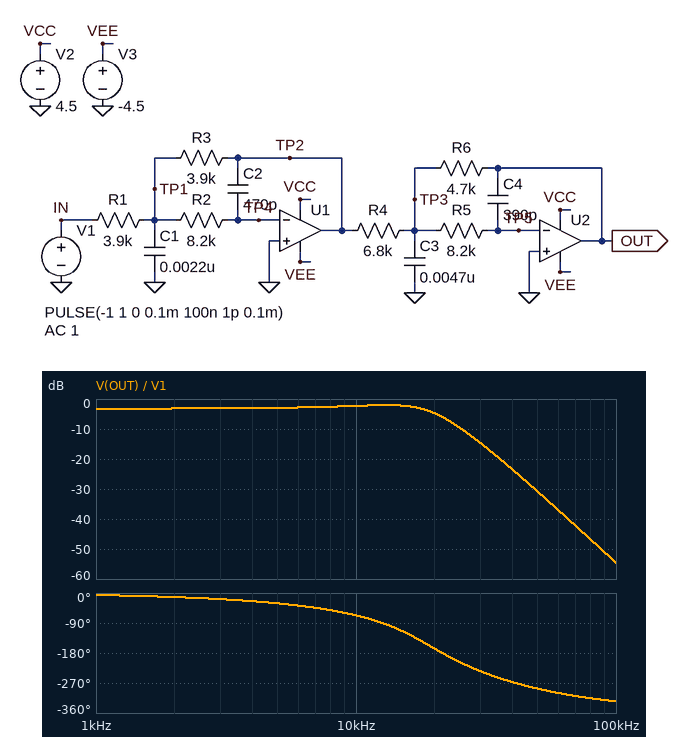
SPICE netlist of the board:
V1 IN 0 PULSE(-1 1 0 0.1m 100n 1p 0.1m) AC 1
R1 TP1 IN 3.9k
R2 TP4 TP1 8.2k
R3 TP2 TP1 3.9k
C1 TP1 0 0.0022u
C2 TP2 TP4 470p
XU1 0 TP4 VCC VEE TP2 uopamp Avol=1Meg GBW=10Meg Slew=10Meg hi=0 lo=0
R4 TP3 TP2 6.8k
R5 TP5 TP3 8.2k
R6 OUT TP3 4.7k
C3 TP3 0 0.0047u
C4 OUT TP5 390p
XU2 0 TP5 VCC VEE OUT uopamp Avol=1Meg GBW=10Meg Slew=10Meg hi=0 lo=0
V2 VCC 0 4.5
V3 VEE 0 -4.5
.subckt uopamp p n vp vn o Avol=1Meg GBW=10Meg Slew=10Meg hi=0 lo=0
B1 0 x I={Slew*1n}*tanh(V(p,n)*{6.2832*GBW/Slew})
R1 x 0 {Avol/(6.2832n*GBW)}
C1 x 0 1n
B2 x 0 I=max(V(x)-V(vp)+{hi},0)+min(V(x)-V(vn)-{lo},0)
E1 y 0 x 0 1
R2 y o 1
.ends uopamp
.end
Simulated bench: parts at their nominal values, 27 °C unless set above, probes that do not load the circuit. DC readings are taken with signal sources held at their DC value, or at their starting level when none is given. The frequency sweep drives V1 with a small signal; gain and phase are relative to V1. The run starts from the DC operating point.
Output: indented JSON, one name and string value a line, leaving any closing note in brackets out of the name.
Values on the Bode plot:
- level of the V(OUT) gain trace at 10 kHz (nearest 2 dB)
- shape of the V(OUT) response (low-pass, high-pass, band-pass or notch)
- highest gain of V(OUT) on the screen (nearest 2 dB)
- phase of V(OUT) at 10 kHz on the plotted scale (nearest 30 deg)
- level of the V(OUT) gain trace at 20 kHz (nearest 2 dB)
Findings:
{
  "level of the V(OUT) gain trace at 10 kHz": "-2 dB",
  "shape of the V(OUT) response": "low-pass",
  "highest gain of V(OUT) on the screen": "-2 dB",
  "phase of V(OUT) at 10 kHz on the plotted scale": "-60 deg",
  "level of the V(OUT) gain trace at 20 kHz": "-4 dB"
}
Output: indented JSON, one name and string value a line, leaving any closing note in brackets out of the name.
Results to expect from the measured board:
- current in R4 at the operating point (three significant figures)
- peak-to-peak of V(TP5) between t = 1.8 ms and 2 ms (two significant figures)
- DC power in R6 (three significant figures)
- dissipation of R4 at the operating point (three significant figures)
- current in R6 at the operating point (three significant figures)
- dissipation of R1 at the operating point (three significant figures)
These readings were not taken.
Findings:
{
  "current in R4 at the operating point": "147 µA",
  "peak-to-peak of V(TP5) between t = 1.8 ms and 2 ms": "1.5 mV",
  "DC power in R6": "102 µW",
  "dissipation of R4 at the operating point": "147 µW",
  "current in R6 at the operating point": "147 µA",
  "dissipation of R1 at the operating point": "256 µW"
}
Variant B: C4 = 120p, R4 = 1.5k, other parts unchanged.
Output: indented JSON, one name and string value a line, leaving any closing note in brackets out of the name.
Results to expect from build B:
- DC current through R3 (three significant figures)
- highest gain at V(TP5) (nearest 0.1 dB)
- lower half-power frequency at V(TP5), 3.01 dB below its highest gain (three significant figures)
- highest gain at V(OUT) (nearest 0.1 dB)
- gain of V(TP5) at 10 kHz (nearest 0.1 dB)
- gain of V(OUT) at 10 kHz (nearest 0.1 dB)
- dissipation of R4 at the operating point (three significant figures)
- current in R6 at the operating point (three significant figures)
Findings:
{
  "DC current through R3": "256 µA",
  "highest gain at V(TP5)": "-44.4 dB",
  "lower half-power frequency at V(TP5), 3.01 dB below its highest gain": "14.1 kHz",
  "highest gain at V(OUT)": "9.9 dB",
  "gain of V(TP5) at 10 kHz": "-50.2 dB",
  "gain of V(OUT) at 10 kHz": "9.8 dB",
  "dissipation of R4 at the operating point": "667 µW",
  "current in R6 at the operating point": "667 µA"
}
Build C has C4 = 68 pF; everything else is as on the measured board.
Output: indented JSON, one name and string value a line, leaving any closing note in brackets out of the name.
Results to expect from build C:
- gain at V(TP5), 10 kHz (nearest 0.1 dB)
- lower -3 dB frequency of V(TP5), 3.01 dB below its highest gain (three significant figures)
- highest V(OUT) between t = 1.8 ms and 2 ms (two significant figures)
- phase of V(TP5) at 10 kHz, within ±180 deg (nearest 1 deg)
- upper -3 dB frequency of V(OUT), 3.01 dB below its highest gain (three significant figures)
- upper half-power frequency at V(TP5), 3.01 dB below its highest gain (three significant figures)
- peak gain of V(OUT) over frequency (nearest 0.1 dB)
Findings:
{
  "gain at V(TP5), 10 kHz": "-63.3 dB",
  "lower -3 dB frequency of V(TP5), 3.01 dB below its highest gain": "31.6 kHz",
  "highest V(OUT) between t = 1.8 ms and 2 ms": "580 mV",
  "phase of V(TP5) at 10 kHz, within ±180 deg": "-130 deg",
  "upper -3 dB frequency of V(OUT), 3.01 dB below its highest gain": "47.7 kHz",
  "upper half-power frequency at V(TP5), 3.01 dB below its highest gain": "49.5 kHz",
  "peak gain of V(OUT) over frequency": "-3.2 dB"
}
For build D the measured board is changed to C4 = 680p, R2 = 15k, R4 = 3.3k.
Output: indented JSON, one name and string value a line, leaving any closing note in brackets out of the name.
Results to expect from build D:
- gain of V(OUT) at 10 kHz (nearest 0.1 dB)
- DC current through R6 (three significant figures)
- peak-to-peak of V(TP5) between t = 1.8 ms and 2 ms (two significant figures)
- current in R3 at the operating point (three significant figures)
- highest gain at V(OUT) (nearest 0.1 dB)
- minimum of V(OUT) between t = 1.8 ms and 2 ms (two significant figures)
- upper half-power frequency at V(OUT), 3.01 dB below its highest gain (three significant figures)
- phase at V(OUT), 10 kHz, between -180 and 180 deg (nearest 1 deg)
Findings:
{
  "gain of V(OUT) at 10 kHz": "-0.3 dB",
  "DC current through R6": "303 µA",
  "peak-to-peak of V(TP5) between t = 1.8 ms and 2 ms": "1.3 mV",
  "current in R3 at the operating point": "256 µA",
  "highest gain at V(OUT)": "3.1 dB",
  "minimum of V(OUT) between t = 1.8 ms and 2 ms": "-590 mV",
  "upper half-power frequency at V(OUT), 3.01 dB below its highest gain": "9.52 kHz",
  "phase at V(OUT), 10 kHz, between -180 and 180 deg": "-117 deg"
}
